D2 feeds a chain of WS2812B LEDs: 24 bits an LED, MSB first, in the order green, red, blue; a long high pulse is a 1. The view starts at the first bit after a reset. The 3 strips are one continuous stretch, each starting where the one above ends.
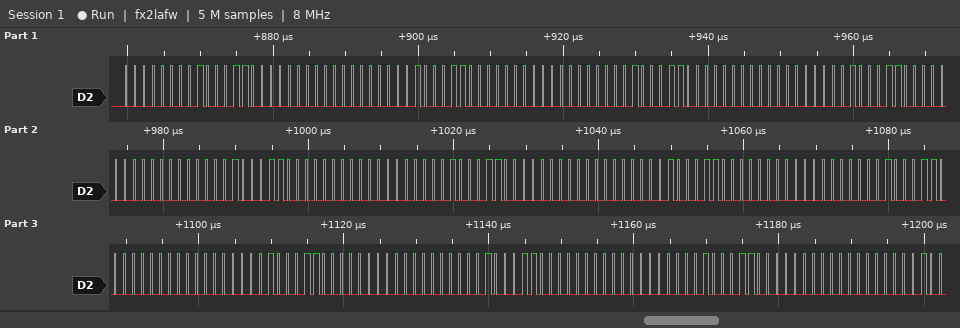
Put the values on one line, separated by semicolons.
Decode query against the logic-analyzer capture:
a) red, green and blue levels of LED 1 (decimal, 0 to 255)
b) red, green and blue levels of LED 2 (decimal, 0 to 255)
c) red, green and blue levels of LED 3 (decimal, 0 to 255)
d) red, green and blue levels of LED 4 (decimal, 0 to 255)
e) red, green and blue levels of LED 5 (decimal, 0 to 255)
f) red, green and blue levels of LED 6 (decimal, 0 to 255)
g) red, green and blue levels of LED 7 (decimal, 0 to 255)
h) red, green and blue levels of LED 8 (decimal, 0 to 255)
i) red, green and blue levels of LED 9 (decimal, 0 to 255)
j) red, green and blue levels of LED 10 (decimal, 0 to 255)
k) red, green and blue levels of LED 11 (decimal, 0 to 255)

140, 0, 0; 140, 0, 0; 140, 0, 0; 140, 0, 0; 140, 0, 0; 140, 0, 0; 140, 0, 0; 140, 0, 0; 140, 0, 0; 140, 0, 0; 140, 0, 0
